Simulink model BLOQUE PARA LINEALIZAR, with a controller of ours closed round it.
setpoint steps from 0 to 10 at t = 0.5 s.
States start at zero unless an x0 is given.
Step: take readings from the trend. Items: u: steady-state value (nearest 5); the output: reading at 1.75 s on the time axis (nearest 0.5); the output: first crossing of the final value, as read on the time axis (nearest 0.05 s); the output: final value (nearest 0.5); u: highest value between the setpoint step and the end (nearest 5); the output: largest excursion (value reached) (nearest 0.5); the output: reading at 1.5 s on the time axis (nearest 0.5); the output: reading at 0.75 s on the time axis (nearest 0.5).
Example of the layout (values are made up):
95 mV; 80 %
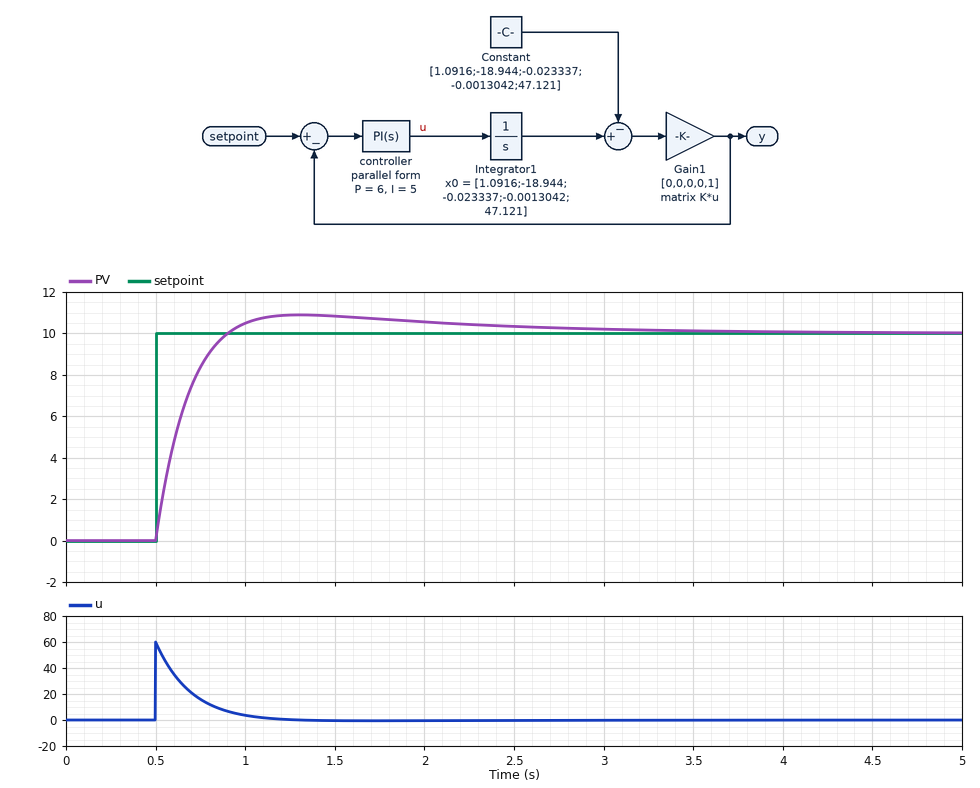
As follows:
0; 10.5; 0.90 s; 10.0; 60; 11.0; 11.0; 8.5
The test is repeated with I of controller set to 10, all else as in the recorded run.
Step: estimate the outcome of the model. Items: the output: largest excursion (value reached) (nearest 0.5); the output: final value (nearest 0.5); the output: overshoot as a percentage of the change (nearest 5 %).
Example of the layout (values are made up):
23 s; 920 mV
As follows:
11.5; 10.0; 15 %
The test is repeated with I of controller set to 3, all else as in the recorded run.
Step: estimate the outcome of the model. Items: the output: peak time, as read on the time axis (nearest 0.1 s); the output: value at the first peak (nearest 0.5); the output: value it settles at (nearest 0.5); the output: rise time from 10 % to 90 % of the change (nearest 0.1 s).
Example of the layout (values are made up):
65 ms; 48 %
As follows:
1.4 s; 10.5; 10.0; 0.3 s
